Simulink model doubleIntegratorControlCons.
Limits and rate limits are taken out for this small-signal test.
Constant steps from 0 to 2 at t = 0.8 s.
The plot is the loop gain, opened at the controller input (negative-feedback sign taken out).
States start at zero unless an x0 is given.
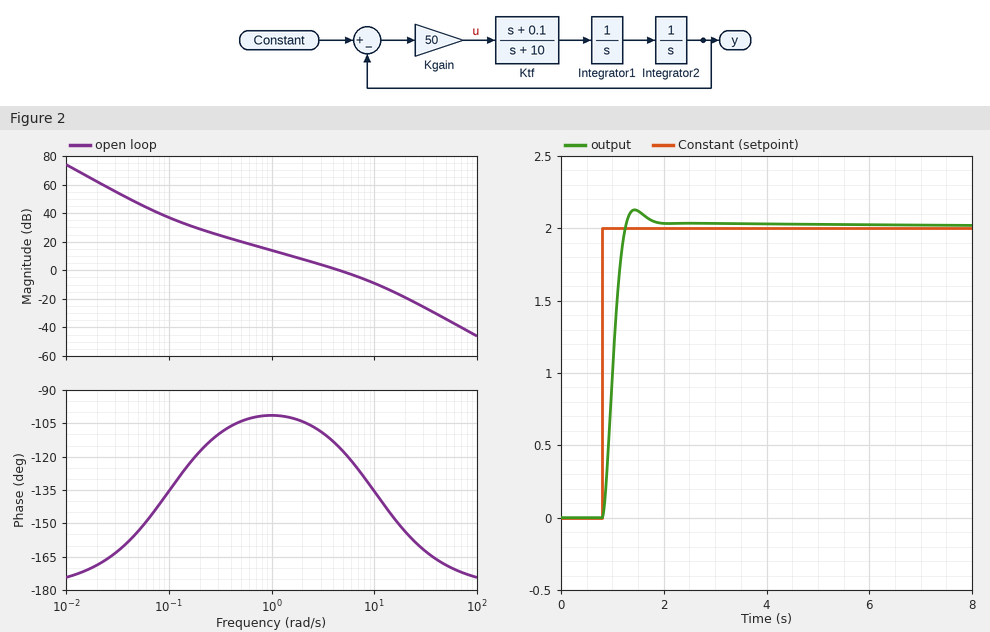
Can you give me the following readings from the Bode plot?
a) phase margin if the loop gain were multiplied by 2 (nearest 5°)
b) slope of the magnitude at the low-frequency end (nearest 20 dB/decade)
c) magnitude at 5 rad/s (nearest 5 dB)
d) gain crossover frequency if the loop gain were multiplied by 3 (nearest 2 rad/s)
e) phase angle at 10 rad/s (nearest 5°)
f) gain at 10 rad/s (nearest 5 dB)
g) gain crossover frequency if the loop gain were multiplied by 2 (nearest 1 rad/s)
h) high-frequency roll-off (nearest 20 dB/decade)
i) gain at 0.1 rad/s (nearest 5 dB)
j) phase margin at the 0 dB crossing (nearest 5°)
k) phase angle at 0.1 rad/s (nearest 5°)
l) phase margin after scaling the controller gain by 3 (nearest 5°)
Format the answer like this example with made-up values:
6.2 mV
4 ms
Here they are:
50°
-40 dB/decade
0 dB
10 rad/s
-135°
-10 dB
8 rad/s
-40 dB/decade
35 dB
65°
-135°
45°
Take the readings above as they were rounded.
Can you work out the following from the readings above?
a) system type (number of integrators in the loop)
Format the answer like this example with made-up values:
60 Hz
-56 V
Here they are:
2
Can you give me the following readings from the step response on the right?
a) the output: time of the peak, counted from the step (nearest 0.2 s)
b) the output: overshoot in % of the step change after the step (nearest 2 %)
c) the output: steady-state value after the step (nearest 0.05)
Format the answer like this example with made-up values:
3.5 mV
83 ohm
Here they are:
0.6 s
6 %
2.00
